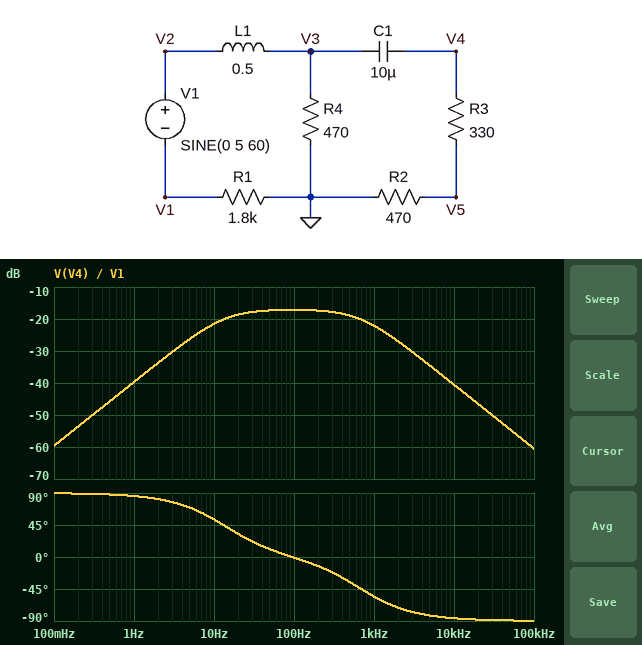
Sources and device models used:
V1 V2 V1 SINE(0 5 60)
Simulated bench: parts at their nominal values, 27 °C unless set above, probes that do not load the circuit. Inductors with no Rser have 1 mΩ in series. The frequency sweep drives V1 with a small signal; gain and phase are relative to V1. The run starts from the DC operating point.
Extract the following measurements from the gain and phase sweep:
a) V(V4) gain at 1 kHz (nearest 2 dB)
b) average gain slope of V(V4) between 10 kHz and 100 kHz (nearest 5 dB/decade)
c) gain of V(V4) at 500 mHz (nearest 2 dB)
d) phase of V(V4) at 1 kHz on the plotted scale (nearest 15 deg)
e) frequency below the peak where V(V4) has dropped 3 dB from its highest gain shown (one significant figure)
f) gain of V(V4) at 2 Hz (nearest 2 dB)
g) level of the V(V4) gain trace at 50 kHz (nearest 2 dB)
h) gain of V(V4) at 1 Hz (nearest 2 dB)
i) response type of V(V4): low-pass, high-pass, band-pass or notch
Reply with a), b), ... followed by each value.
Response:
a) -22 dB
b) -20 dB/decade
c) -46 dB
d) -60 deg
e) 10 Hz
f) -34 dB
g) -54 dB
h) -40 dB
i) band-pass
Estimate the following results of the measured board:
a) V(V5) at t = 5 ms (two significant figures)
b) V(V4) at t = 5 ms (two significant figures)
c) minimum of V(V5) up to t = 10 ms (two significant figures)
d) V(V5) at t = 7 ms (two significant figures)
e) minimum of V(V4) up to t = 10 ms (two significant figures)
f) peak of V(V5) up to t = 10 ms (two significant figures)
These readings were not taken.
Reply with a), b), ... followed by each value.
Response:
a) 300 mV
b) 520 mV
c) -320 mV
d) 96 mV
e) -540 mV
f) 340 mV
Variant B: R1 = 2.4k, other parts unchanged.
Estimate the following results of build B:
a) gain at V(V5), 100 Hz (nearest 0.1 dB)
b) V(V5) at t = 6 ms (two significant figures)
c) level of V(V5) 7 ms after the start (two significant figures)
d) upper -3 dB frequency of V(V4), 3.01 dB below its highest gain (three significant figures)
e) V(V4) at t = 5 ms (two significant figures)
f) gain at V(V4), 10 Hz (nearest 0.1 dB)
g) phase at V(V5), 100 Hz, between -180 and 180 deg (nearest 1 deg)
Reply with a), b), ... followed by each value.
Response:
a) -23.9 dB
b) 170 mV
c) 70 mV
d) 884 Hz
e) 400 mV
f) -23.6 dB
g) 1 deg
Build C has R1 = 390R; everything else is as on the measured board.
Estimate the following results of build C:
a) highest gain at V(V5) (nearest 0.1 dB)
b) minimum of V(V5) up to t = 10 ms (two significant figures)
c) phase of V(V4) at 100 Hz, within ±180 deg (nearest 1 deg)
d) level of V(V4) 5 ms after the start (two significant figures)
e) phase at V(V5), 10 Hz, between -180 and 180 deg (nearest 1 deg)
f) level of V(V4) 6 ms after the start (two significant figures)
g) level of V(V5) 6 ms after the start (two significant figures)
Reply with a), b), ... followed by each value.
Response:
a) -12.4 dB
b) -820 mV
c) -16 deg
d) 1.6 V
e) 55 deg
f) 1.3 V
g) 740 mV
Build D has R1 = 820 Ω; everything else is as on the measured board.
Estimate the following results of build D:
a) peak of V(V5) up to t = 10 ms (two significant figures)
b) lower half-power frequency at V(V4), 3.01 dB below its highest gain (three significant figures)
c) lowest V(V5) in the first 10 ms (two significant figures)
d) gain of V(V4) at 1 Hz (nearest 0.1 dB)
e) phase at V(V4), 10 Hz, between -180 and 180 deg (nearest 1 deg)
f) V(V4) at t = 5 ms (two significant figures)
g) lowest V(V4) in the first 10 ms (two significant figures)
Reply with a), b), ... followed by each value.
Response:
a) 620 mV
b) 13.5 Hz
c) -560 mV
d) -34.8 dB
e) 54 deg
f) 980 mV
g) -950 mV
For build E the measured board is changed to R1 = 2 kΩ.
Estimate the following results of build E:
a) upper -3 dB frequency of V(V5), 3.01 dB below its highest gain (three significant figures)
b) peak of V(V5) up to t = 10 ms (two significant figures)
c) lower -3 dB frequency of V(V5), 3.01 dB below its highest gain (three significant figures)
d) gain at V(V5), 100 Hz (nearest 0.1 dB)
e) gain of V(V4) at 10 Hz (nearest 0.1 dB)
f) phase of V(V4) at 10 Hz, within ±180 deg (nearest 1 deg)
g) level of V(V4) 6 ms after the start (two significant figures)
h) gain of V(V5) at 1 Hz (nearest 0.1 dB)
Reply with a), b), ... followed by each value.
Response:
a) 756 Hz
b) 310 mV
c) 13.0 Hz
d) -22.6 dB
e) -22.3 dB
f) 53 deg
g) 340 mV
h) -45.0 dB
